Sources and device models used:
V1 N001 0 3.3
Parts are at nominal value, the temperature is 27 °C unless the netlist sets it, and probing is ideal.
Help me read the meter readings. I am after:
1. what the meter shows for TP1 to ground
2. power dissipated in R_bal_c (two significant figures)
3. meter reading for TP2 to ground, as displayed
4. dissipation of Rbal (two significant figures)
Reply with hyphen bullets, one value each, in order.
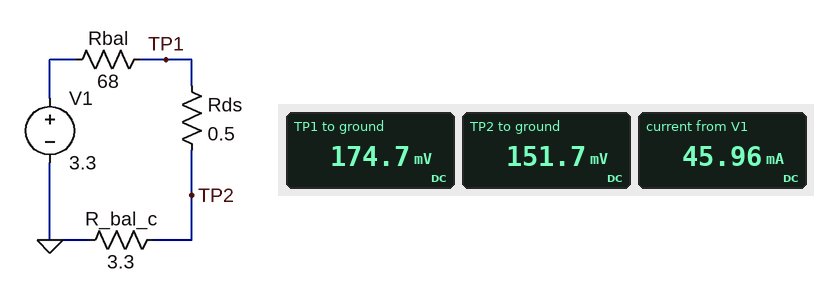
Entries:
- 174.7 mV
- 7.0 mW
- 151.7 mV
- 140 mW
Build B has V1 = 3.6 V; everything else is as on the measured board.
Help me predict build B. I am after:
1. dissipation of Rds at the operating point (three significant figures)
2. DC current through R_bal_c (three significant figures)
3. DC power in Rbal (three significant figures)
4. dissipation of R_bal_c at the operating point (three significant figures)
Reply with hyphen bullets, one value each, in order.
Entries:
- 1.26 mW
- 50.1 mA
- 171 mW
- 8.30 mW
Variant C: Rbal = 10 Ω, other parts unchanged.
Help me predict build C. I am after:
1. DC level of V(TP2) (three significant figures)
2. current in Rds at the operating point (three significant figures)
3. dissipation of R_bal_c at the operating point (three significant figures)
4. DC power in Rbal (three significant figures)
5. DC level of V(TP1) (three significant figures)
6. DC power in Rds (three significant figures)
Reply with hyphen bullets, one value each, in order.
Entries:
- 789 mV
- 239 mA
- 189 mW
- 572 mW
- 909 mV
- 28.6 mW
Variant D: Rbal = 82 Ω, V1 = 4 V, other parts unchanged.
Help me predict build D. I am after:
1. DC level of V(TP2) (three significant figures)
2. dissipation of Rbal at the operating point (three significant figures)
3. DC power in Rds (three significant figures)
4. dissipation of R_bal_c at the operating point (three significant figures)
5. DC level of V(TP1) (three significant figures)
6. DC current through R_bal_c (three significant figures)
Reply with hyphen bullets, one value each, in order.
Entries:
- 154 mV
- 178 mW
- 1.09 mW
- 7.17 mW
- 177 mV
- 46.6 mA
